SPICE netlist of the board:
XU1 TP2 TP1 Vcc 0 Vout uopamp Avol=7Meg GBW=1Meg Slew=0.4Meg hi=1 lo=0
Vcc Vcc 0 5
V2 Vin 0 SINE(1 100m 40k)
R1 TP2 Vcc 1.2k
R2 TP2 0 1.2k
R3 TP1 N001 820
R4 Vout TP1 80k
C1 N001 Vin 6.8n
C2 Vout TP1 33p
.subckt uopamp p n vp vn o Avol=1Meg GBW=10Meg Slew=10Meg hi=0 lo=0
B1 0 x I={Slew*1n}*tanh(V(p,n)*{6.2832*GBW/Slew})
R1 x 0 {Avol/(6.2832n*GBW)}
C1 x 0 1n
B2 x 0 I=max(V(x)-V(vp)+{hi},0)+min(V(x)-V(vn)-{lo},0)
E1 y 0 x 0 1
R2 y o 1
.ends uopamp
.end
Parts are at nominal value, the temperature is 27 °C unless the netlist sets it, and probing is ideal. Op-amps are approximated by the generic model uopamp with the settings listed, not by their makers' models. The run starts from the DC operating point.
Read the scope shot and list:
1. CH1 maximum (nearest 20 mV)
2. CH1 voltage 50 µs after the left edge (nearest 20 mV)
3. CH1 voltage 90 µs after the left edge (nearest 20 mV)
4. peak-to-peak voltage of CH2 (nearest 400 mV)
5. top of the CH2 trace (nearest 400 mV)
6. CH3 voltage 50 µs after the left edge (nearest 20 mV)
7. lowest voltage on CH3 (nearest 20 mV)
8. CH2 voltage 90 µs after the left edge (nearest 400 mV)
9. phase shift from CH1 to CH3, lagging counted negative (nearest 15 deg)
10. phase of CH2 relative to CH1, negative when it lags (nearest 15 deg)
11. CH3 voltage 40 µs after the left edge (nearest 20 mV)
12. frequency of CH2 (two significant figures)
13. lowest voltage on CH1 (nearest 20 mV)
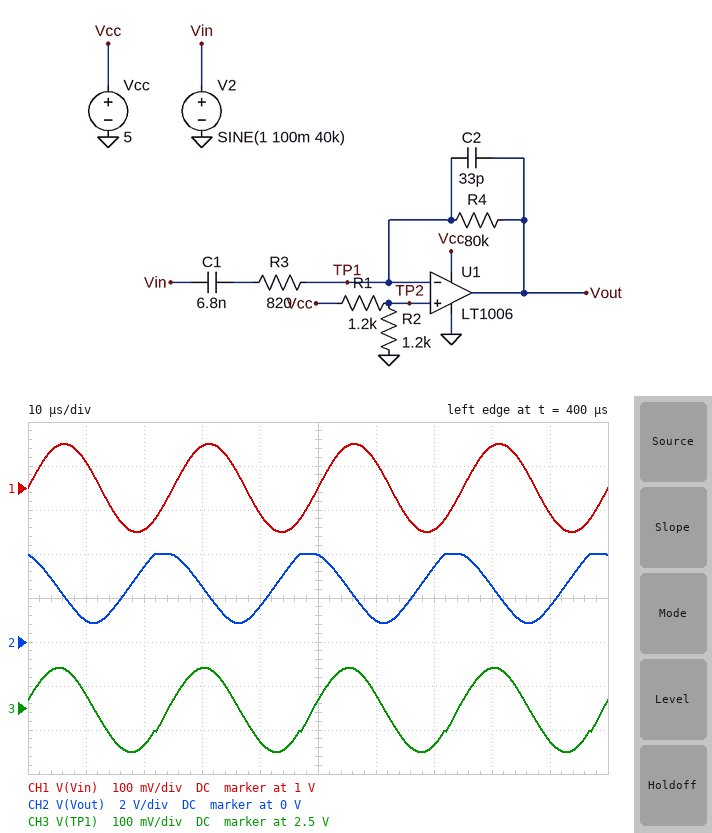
1.10 V
1.00 V
940 mV
3.2 V
4.0 V
2.52 V
2.40 V
1.6 V
15 deg
105 deg
2.42 V
40 kHz
900 mV
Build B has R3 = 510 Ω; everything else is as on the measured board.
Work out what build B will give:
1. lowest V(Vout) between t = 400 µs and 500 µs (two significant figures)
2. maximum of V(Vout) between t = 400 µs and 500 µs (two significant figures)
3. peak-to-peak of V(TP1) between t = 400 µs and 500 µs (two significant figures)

810 mV
4.0 V
200 mV
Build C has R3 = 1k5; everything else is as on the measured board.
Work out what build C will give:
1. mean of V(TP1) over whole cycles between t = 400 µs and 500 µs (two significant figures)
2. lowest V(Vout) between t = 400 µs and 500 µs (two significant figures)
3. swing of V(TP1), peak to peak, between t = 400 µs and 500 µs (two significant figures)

2.5 V
950 mV
170 mV
